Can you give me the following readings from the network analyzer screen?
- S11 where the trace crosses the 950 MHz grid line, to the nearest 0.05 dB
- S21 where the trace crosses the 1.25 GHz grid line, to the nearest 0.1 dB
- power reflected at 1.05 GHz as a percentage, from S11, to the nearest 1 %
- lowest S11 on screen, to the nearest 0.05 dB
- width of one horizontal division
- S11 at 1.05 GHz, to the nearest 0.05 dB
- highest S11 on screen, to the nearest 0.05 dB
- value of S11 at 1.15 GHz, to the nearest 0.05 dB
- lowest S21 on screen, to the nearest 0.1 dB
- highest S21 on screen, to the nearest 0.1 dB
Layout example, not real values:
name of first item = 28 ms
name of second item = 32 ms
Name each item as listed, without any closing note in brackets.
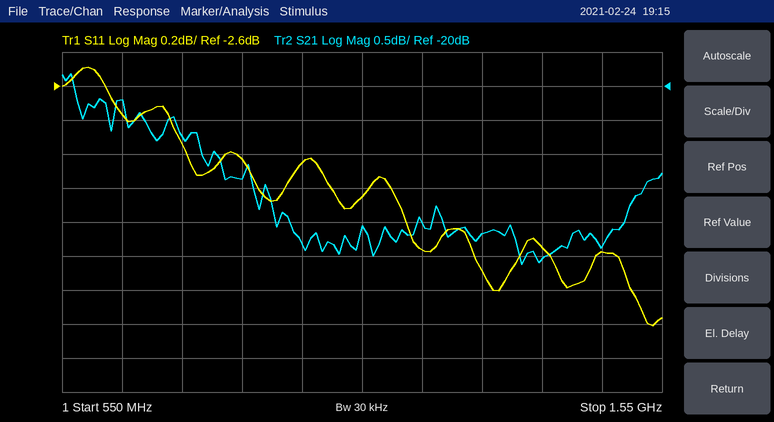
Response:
S11 where the trace crosses the 950 MHz grid line, to the nearest 0.05 dB = -3.05 dB
S21 where the trace crosses the 1.25 GHz grid line, to the nearest 0.1 dB = -22.2 dB
power reflected at 1.05 GHz as a percentage, from S11, to the nearest 1 % = 47 %
lowest S11 on screen, to the nearest 0.05 dB = -4.00 dB
width of one horizontal division = 100 MHz
S11 at 1.05 GHz, to the nearest 0.05 dB = -3.25 dB
highest S11 on screen, to the nearest 0.05 dB = -2.50 dB
value of S11 at 1.15 GHz, to the nearest 0.05 dB = -3.55 dB
lowest S21 on screen, to the nearest 0.1 dB = -22.6 dB
highest S21 on screen, to the nearest 0.1 dB = -19.8 dB
